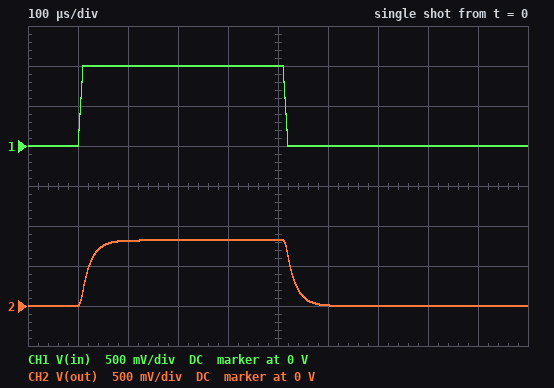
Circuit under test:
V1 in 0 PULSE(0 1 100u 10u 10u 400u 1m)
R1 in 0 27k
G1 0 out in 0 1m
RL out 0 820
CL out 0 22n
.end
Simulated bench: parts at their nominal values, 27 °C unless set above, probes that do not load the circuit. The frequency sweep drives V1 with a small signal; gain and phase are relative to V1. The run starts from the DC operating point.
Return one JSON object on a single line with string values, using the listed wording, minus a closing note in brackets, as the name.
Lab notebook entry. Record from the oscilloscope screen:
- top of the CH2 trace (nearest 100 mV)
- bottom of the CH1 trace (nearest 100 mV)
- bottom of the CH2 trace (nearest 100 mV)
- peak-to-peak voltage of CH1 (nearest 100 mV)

{"top of the CH2 trace": "800 mV", "bottom of the CH1 trace": "0 V", "bottom of the CH2 trace": "0 V", "peak-to-peak voltage of CH1": "1.0 V"}
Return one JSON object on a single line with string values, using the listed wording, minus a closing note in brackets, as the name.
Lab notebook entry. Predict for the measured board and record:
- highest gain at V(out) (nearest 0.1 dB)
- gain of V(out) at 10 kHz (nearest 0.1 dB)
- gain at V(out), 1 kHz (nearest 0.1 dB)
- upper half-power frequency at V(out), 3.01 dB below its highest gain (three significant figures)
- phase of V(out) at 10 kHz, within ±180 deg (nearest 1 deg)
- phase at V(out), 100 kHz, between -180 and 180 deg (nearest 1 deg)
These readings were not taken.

{"highest gain at V(out)": "-1.7 dB", "gain of V(out) at 10 kHz": "-5.3 dB", "gain at V(out), 1 kHz": "-1.8 dB", "upper half-power frequency at V(out), 3.01 dB below its highest gain": "8.82 kHz", "phase of V(out) at 10 kHz, within ±180 deg": "-49 deg", "phase at V(out), 100 kHz, between -180 and 180 deg": "-85 deg"}
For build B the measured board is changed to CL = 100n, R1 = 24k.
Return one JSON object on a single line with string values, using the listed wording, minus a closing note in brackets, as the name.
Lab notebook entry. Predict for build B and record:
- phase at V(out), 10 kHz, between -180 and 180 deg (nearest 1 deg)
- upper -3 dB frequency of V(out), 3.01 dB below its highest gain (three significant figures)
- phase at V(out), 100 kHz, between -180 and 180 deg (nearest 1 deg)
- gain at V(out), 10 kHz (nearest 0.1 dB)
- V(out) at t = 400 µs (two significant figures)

{"phase at V(out), 10 kHz, between -180 and 180 deg": "-79 deg", "upper -3 dB frequency of V(out), 3.01 dB below its highest gain": "1.94 kHz", "phase at V(out), 100 kHz, between -180 and 180 deg": "-89 deg", "gain at V(out), 10 kHz": "-16.1 dB", "V(out) at t = 400 µs": "800 mV"}
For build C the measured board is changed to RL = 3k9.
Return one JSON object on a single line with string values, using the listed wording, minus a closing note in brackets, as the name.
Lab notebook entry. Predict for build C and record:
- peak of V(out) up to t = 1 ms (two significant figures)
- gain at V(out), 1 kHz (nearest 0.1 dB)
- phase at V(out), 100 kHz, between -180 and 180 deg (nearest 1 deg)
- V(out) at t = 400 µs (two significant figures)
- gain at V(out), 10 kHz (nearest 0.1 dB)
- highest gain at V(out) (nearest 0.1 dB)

{"peak of V(out) up to t = 1 ms": "3.9 V", "gain at V(out), 1 kHz": "10.7 dB", "phase at V(out), 100 kHz, between -180 and 180 deg": "-89 deg", "V(out) at t = 400 µs": "3.8 V", "gain at V(out), 10 kHz": "-3.0 dB", "highest gain at V(out)": "11.8 dB"}
